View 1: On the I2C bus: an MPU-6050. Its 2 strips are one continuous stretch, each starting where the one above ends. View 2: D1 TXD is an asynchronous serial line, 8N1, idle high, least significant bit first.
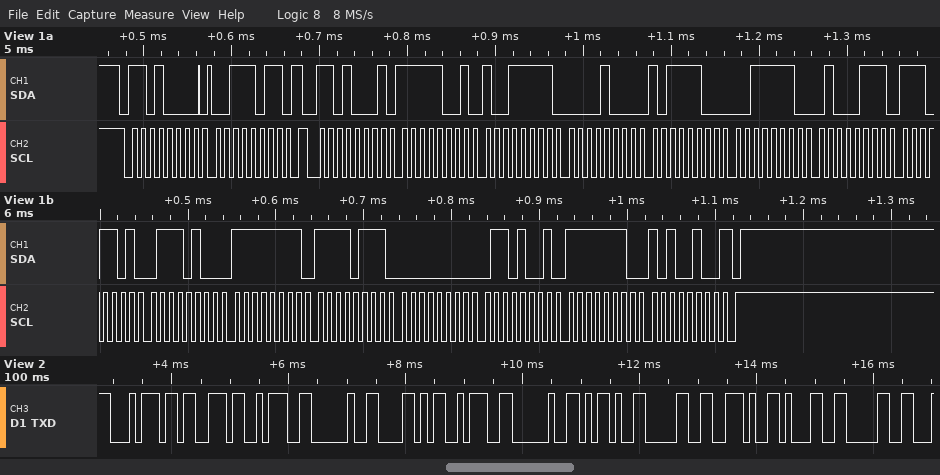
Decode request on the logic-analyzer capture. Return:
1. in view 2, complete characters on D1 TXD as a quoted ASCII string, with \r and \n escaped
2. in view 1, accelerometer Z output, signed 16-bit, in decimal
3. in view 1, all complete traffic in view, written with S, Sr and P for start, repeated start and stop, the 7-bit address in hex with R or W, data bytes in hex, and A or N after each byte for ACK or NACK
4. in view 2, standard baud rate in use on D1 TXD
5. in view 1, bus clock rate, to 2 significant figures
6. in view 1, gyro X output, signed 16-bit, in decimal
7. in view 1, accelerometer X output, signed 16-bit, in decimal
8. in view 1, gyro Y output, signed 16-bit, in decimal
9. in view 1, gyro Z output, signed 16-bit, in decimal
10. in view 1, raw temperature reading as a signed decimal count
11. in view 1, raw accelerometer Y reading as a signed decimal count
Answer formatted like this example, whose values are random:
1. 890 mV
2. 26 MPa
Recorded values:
1. "ts: X: -0.10"
2. 15943
3. S 68W A 3B A Sr 68R A F9 A 9F A 08 A BC A 3E A 47 A ED A 74 A FF A F7 A 00 A 69 A FE A A4 N P
4. 9600 baud
5. 100 kHz
6. -9
7. -1633
8. 105
9. -348
10. -4748
11. 2236
